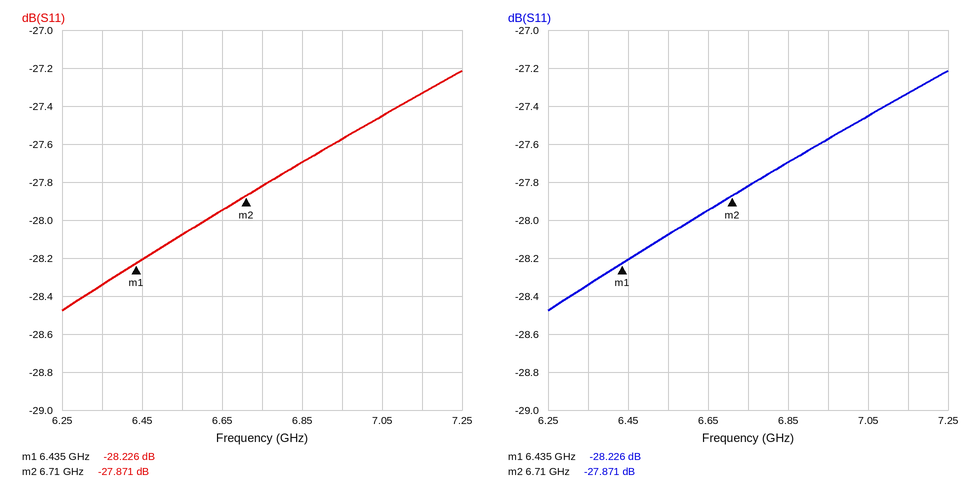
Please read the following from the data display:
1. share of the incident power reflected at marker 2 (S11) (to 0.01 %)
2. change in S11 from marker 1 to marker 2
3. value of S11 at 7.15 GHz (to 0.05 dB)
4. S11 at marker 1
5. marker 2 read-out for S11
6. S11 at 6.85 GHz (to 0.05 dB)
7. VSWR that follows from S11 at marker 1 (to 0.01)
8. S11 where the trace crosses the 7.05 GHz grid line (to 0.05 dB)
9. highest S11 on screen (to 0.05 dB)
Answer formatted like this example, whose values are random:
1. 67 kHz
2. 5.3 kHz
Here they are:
1. 0.16 %
2. 0.355 dB
3. -27.35 dB
4. -28.226 dB
5. -27.871 dB
6. -27.70 dB
7. 1.08
8. -27.45 dB
9. -27.20 dB
